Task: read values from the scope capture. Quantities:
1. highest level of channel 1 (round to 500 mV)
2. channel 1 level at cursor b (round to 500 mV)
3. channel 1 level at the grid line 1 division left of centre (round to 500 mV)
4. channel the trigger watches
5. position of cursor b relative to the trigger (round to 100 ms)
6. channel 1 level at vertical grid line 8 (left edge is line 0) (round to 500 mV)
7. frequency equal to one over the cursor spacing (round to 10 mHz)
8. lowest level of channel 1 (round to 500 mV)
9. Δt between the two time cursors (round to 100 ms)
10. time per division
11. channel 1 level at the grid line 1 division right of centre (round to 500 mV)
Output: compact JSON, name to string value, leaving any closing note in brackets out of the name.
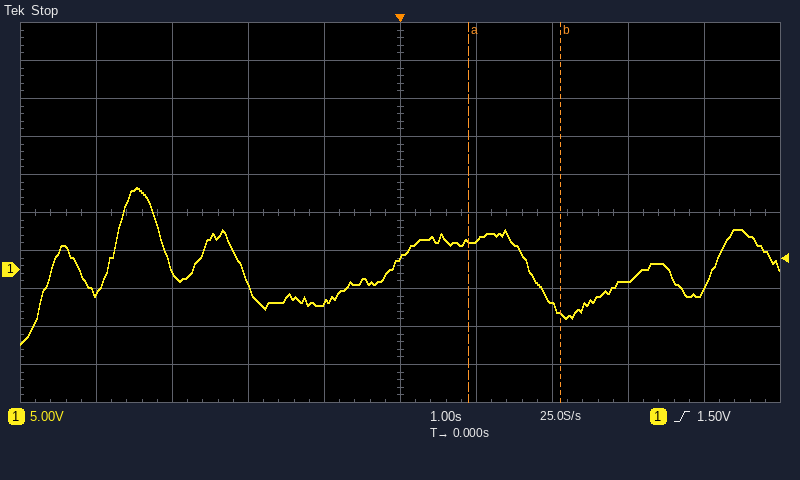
{"highest level of channel 1": "11.0 V", "channel 1 level at cursor b": "-6.0 V", "channel 1 level at the grid line 1 division left of centre": "-4.5 V", "channel the trigger watches": "channel 1", "position of cursor b relative to the trigger": "+2.1 s", "channel 1 level at vertical grid line 8 (left edge is line 0)": "-1.5 V", "frequency equal to one over the cursor spacing": "830 mHz", "lowest level of channel 1": "-10.0 V", "Δt between the two time cursors": "1.2 s", "time per division": "1 s", "channel 1 level at the grid line 1 division right of centre": "4.0 V"}
